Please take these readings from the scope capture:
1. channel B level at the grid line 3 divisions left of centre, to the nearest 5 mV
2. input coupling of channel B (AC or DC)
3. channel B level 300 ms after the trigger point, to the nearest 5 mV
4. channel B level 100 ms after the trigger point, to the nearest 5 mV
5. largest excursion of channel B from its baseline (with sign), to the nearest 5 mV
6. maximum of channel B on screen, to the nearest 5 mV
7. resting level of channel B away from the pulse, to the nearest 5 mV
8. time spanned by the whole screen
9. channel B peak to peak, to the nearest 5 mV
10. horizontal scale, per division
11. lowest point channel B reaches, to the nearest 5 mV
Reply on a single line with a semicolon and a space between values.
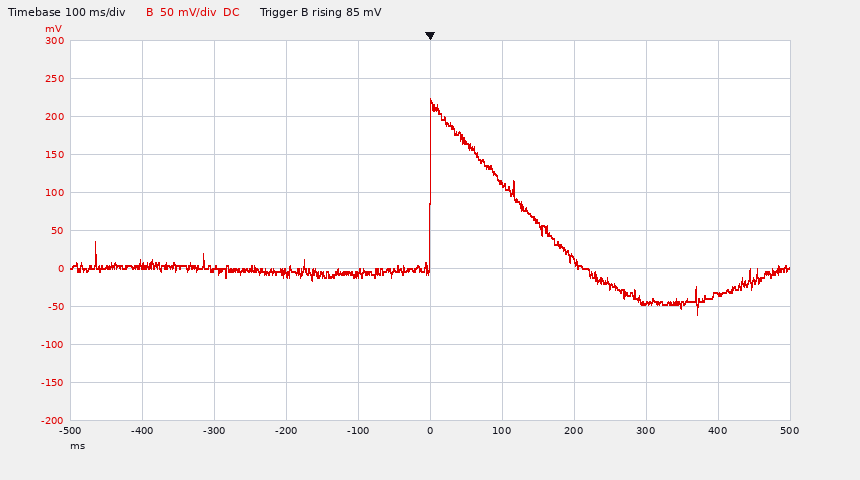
0 mV; DC; -45 mV; 110 mV; +225 mV; 225 mV; 0 mV; 1 s; 285 mV; 100 ms; -60 mV
